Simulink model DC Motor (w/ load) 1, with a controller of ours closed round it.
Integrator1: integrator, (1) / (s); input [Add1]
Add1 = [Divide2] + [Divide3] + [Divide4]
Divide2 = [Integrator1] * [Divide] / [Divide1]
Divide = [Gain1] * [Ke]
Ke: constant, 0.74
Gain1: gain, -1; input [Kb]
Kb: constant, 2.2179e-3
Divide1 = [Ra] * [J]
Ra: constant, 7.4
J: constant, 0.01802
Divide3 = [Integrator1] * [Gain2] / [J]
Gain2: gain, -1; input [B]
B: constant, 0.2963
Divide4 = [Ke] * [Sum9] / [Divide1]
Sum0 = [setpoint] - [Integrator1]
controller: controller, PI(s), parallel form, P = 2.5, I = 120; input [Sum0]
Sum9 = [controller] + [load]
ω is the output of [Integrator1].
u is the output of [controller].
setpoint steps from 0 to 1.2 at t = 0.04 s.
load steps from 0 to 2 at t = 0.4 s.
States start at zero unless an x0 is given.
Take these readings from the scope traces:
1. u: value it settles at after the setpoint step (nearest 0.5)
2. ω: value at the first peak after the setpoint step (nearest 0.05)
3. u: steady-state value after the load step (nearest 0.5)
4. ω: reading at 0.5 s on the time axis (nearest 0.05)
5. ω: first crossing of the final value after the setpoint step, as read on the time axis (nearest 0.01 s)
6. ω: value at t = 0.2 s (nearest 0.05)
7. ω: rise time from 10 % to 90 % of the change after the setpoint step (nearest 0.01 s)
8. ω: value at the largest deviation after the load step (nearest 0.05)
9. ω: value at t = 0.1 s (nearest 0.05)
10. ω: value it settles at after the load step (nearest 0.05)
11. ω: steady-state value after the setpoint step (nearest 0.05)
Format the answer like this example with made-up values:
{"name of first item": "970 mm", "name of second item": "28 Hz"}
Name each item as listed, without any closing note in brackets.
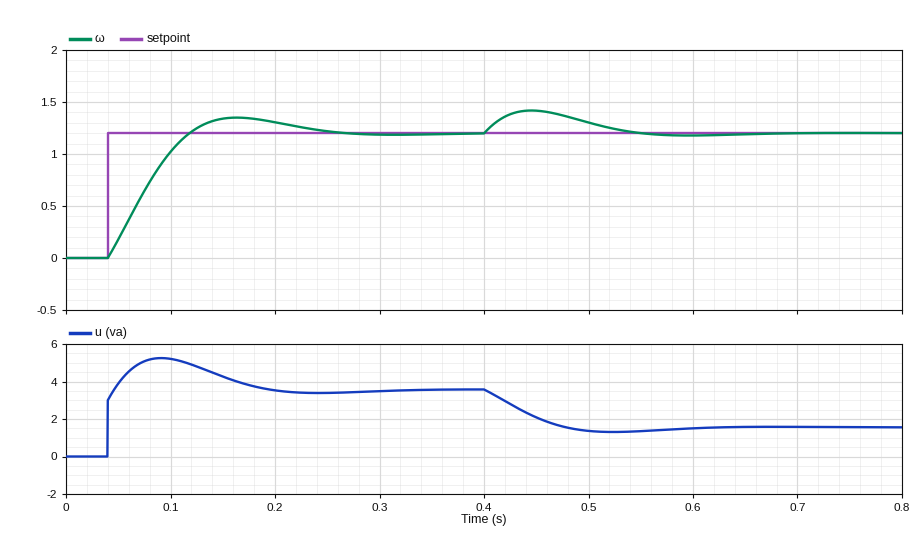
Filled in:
{"u: value it settles at after the setpoint step": "3.5", "ω: value at the first peak after the setpoint step": "1.35", "u: steady-state value after the load step": "1.5", "ω: reading at 0.5 s on the time axis": "1.30", "ω: first crossing of the final value after the setpoint step, as read on the time axis": "0.12 s", "ω: value at t = 0.2 s": "1.30", "ω: rise time from 10 % to 90 % of the change after the setpoint step": "0.06 s", "ω: value at the largest deviation after the load step": "1.40", "ω: value at t = 0.1 s": "1.00", "ω: value it settles at after the load step": "1.20", "ω: steady-state value after the setpoint step": "1.20"}
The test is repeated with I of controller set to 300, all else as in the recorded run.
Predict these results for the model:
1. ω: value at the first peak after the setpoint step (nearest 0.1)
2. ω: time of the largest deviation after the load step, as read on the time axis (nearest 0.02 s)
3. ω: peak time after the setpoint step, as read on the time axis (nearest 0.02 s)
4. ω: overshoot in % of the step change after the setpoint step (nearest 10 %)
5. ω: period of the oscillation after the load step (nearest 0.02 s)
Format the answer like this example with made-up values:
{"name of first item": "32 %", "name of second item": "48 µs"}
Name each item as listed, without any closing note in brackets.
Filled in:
{"ω: value at the first peak after the setpoint step": "1.6", "ω: time of the largest deviation after the load step, as read on the time axis": "0.44 s", "ω: peak time after the setpoint step, as read on the time axis": "0.12 s", "ω: overshoot in % of the step change after the setpoint step": "30 %", "ω: period of the oscillation after the load step": "0.16 s"}
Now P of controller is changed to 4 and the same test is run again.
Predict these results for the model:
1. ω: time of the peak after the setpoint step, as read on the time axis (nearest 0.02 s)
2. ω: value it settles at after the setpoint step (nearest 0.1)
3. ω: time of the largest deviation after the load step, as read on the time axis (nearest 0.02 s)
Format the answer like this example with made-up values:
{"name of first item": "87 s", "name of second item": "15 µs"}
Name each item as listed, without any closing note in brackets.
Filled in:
{"ω: time of the peak after the setpoint step, as read on the time axis": "0.16 s", "ω: value it settles at after the setpoint step": "1.2", "ω: time of the largest deviation after the load step, as read on the time axis": "0.44 s"}
